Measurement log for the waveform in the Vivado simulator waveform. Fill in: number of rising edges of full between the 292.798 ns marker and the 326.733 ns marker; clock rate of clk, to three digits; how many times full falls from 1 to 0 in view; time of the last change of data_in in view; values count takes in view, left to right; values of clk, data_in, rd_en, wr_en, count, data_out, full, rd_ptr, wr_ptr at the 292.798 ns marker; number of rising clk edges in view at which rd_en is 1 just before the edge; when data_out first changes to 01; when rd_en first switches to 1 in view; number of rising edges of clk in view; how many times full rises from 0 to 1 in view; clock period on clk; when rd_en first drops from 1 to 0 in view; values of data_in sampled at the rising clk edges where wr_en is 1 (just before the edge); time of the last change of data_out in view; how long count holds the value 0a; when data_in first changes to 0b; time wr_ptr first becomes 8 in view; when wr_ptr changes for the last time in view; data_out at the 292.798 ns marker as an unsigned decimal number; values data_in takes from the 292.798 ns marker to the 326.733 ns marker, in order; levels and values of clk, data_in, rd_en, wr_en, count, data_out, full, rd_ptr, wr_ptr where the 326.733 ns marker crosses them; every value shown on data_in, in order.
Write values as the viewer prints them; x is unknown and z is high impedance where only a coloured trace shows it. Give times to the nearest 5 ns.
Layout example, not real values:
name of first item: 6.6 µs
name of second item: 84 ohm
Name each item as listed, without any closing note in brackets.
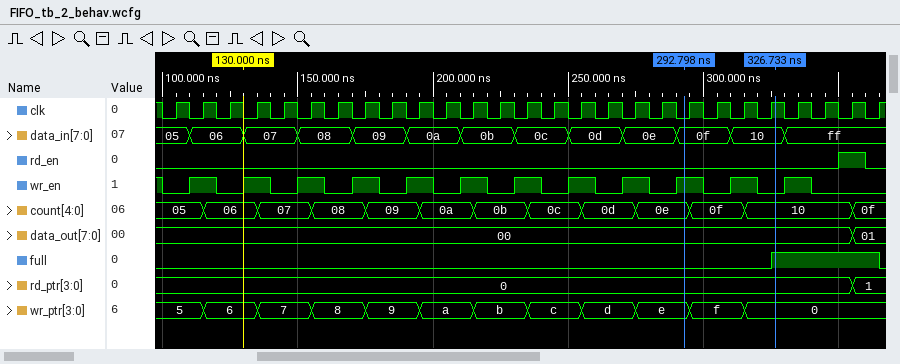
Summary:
number of rising edges of full between the 292.798 ns marker and the 326.733 ns marker: 1
clock rate of clk, to three digits: 100 MHz
how many times full falls from 1 to 0 in view: 1
time of the last change of data_in in view: 330 ns
values count takes in view, left to right: 05, 06, 07, 08, 09, 0a, 0b, 0c, 0d, 0e, 0f, 10, 0f
values of clk, data_in, rd_en, wr_en, count, data_out, full, rd_ptr, wr_ptr at the 292.798 ns marker: clk=0, data_in=0f, rd_en=0, wr_en=1, count=0e, data_out=00, full=0, rd_ptr=0, wr_ptr=e
number of rising clk edges in view at which rd_en is 1 just before the edge: 1
when data_out first changes to 01: 355 ns
when rd_en first switches to 1 in view: 350 ns
number of rising edges of clk in view: 27
how many times full rises from 0 to 1 in view: 1
clock period on clk: 10 ns
when rd_en first drops from 1 to 0 in view: 360 ns
values of data_in sampled at the rising clk edges where wr_en is 1: 06, 07, 08, 09, 0a, 0b, 0c, 0d, 0e, 0f, 10, ff
time of the last change of data_out in view: 355 ns
how long count holds the value 0a: 20 ns
when data_in first changes to 0b: 210 ns
time wr_ptr first becomes 8 in view: 155 ns
when wr_ptr changes for the last time in view: 315 ns
data_out at the 292.798 ns marker as an unsigned decimal number: 0
values data_in takes from the 292.798 ns marker to the 326.733 ns marker, in order: 0f, 10
levels and values of clk, data_in, rd_en, wr_en, count, data_out, full, rd_ptr, wr_ptr where the 326.733 ns marker crosses them: clk=1, data_in=10, rd_en=0, wr_en=0, count=10, data_out=00, full=1, rd_ptr=0, wr_ptr=0
every value shown on data_in, in order: 05, 06, 07, 08, 09, 0a, 0b, 0c, 0d, 0e, 0f, 10, ff
